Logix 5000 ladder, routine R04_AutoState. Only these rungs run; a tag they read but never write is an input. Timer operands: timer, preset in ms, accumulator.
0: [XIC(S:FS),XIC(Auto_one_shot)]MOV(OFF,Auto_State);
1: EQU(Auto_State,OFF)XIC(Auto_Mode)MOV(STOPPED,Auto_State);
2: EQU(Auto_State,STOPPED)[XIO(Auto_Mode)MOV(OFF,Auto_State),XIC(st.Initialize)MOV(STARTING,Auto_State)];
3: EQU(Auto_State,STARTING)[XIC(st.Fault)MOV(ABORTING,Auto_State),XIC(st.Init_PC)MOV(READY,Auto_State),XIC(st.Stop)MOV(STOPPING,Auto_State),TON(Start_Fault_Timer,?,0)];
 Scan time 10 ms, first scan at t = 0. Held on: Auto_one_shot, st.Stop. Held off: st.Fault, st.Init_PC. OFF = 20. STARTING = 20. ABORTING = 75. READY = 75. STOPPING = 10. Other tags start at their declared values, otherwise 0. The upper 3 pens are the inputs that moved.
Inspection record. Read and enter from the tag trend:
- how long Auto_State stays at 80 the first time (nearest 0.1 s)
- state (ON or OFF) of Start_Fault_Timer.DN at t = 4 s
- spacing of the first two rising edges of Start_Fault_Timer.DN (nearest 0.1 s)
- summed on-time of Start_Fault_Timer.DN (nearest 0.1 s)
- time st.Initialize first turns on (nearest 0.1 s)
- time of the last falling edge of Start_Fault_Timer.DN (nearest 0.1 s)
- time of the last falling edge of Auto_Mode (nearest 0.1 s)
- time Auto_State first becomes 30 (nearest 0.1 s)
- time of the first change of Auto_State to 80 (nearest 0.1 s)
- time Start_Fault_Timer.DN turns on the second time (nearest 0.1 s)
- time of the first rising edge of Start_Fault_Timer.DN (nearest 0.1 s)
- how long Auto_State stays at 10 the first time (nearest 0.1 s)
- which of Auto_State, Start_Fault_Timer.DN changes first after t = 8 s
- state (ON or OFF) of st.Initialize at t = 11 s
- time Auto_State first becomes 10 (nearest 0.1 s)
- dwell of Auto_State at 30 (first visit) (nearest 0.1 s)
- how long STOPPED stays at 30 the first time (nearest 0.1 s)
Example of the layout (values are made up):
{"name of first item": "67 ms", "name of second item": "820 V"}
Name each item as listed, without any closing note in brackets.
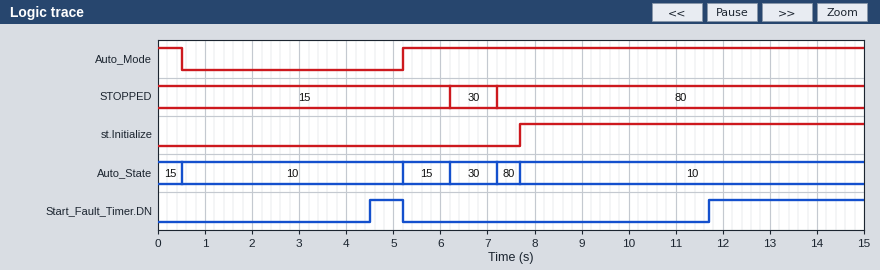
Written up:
{"how long Auto_State stays at 80 the first time": "0.5 s", "state (ON or OFF) of Start_Fault_Timer.DN at t = 4 s": "OFF", "spacing of the first two rising edges of Start_Fault_Timer.DN": "7.2 s", "summed on-time of Start_Fault_Timer.DN": "4.0 s", "time st.Initialize first turns on": "7.7 s", "time of the last falling edge of Start_Fault_Timer.DN": "5.2 s", "time of the last falling edge of Auto_Mode": "0.5 s", "time Auto_State first becomes 30": "6.2 s", "time of the first change of Auto_State to 80": "7.2 s", "time Start_Fault_Timer.DN turns on the second time": "11.7 s", "time of the first rising edge of Start_Fault_Timer.DN": "4.5 s", "how long Auto_State stays at 10 the first time": "4.7 s", "which of Auto_State, Start_Fault_Timer.DN changes first after t = 8 s": "Start_Fault_Timer.DN", "state (ON or OFF) of st.Initialize at t = 11 s": "ON", "time Auto_State first becomes 10": "0.5 s", "dwell of Auto_State at 30 (first visit)": "1.0 s", "how long STOPPED stays at 30 the first time": "1.0 s"}
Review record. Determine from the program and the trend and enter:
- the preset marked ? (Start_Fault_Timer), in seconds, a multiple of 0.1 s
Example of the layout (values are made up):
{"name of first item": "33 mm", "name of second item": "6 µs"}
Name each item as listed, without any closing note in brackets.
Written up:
{"the preset marked ? (Start_Fault_Timer), in seconds, a multiple of 0.1 s": "4.0 s"}
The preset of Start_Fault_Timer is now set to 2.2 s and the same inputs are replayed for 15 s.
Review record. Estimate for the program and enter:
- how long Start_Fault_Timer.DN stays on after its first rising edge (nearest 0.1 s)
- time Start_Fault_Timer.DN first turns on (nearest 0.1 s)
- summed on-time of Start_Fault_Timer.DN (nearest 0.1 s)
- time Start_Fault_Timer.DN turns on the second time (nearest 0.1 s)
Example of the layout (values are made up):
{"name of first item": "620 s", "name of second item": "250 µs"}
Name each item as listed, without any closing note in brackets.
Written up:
{"how long Start_Fault_Timer.DN stays on after its first rising edge": "2.5 s", "time Start_Fault_Timer.DN first turns on": "2.7 s", "summed on-time of Start_Fault_Timer.DN": "7.6 s", "time Start_Fault_Timer.DN turns on the second time": "9.9 s"}
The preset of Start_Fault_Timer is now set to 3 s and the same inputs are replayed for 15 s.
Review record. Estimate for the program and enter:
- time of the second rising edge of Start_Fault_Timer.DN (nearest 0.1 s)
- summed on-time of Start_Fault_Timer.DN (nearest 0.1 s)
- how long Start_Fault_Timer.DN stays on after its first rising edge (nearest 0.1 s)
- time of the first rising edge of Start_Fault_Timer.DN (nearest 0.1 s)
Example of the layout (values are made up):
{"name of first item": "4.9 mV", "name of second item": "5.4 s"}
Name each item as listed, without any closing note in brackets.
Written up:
{"time of the second rising edge of Start_Fault_Timer.DN": "10.7 s", "summed on-time of Start_Fault_Timer.DN": "6.0 s", "how long Start_Fault_Timer.DN stays on after its first rising edge": "1.7 s", "time of the first rising edge of Start_Fault_Timer.DN": "3.5 s"}
